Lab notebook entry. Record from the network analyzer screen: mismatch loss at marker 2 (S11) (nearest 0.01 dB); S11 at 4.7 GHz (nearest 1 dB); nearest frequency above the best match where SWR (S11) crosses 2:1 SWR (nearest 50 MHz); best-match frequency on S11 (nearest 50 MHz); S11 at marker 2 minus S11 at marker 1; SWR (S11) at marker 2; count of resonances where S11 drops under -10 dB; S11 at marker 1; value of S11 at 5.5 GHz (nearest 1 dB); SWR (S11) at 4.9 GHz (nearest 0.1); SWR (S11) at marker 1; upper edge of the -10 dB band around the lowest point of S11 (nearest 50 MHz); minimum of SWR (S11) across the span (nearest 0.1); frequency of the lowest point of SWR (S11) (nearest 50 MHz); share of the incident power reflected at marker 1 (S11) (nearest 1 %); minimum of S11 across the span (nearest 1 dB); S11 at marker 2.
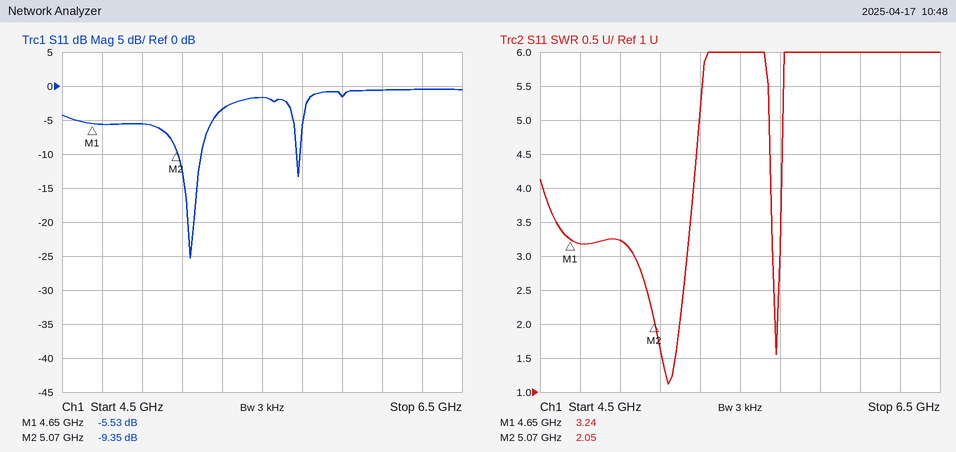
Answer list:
0.54 dB
-6 dB
5.20 GHz
5.15 GHz
-3.82 dB
2.05
2
-5.53 dB
-2 dB
3.2
3.24
5.20 GHz
1.1
5.15 GHz
28 %
-25 dB
-9.35 dB
